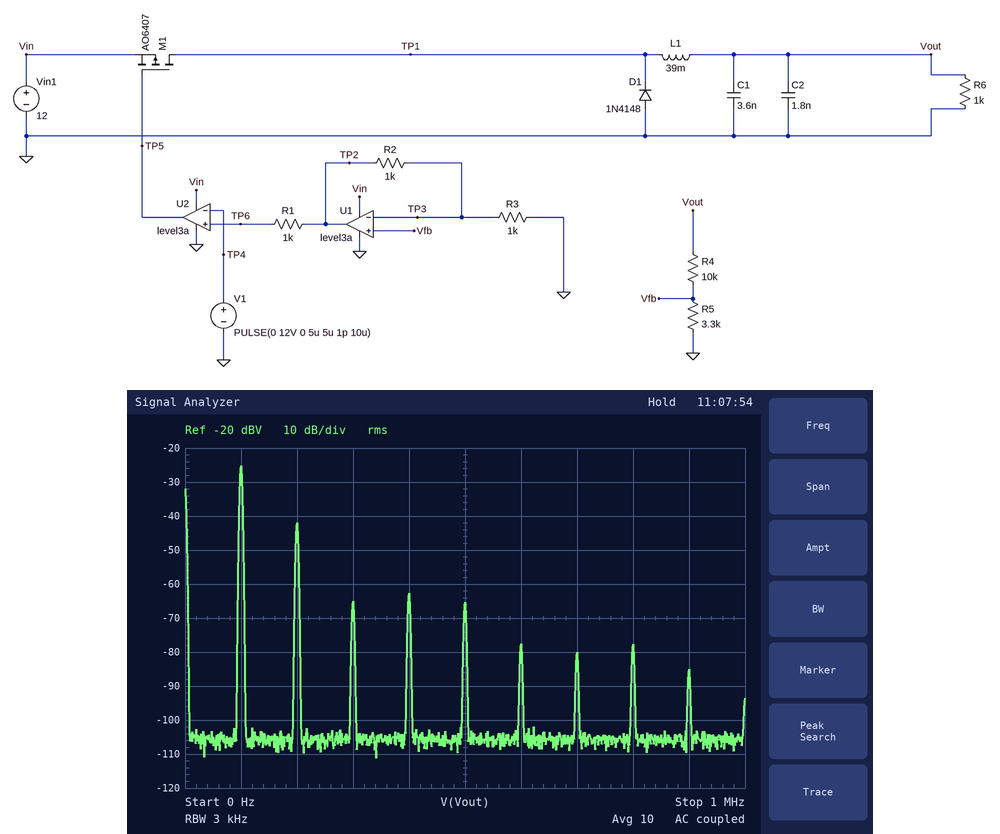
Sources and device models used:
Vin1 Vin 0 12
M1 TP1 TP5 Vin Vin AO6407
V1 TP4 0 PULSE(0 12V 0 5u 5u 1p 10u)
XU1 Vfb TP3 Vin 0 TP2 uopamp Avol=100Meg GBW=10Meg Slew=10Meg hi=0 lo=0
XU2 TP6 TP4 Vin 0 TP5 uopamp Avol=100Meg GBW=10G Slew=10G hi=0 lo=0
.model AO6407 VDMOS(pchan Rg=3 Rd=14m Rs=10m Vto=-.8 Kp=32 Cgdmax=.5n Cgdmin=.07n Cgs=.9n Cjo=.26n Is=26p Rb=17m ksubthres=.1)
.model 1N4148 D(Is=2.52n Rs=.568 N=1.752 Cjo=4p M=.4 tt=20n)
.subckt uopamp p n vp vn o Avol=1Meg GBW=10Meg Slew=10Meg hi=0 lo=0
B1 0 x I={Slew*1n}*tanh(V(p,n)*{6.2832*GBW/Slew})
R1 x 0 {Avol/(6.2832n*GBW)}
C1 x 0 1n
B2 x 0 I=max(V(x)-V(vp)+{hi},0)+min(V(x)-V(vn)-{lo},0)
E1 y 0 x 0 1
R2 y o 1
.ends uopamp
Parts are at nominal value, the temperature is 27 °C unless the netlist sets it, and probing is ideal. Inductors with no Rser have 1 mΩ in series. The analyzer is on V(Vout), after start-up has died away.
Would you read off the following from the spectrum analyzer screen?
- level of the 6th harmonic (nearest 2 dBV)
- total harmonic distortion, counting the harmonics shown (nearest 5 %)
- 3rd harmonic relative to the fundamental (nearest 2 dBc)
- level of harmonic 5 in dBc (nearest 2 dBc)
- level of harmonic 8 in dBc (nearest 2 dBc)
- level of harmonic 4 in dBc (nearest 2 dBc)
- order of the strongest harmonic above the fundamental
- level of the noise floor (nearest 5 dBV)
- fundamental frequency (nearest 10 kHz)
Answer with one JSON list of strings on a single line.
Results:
["-78 dBV", "15 %", "-40 dBc", "-40 dBc", "-52 dBc", "-38 dBc", "2", "-105 dBV", "100 kHz"]
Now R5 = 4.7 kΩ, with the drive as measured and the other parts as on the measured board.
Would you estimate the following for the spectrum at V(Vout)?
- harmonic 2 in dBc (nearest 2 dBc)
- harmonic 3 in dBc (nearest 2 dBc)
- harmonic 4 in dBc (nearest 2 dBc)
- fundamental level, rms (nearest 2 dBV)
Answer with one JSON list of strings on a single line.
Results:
["-20 dBc", "-38 dBc", "-36 dBc", "-24 dBV"]
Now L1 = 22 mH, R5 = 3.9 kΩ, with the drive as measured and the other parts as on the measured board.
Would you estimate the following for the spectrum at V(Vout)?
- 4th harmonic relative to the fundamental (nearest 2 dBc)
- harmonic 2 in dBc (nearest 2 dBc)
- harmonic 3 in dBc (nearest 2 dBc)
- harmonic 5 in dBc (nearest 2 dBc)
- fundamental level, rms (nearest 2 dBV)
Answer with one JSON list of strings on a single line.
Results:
["-36 dBc", "-18 dBc", "-54 dBc", "-42 dBc", "-20 dBV"]
